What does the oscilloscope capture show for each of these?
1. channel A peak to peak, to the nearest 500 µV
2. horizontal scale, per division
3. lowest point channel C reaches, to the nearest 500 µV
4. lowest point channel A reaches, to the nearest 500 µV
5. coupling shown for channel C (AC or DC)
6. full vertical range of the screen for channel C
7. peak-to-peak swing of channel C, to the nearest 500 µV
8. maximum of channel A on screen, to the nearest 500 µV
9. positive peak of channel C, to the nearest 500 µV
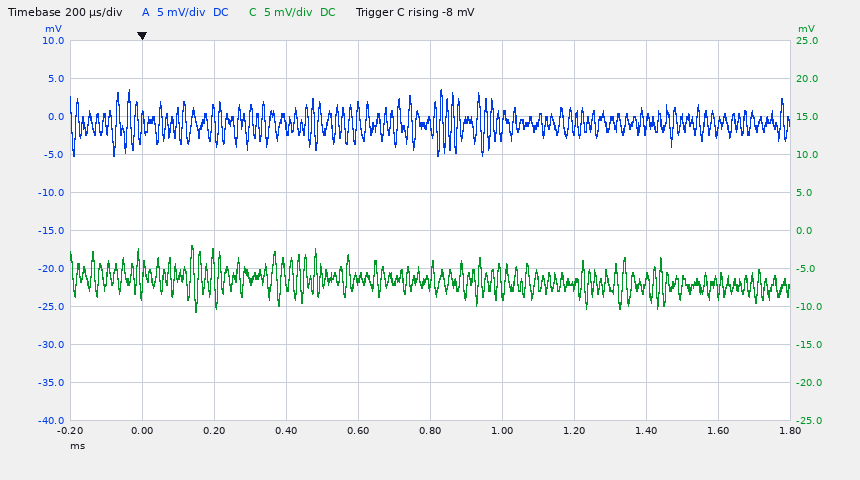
8.5 mV
200 µs
-10.5 mV
-5.0 mV
DC
50 mV
8.5 mV
3.5 mV
-2.0 mV
